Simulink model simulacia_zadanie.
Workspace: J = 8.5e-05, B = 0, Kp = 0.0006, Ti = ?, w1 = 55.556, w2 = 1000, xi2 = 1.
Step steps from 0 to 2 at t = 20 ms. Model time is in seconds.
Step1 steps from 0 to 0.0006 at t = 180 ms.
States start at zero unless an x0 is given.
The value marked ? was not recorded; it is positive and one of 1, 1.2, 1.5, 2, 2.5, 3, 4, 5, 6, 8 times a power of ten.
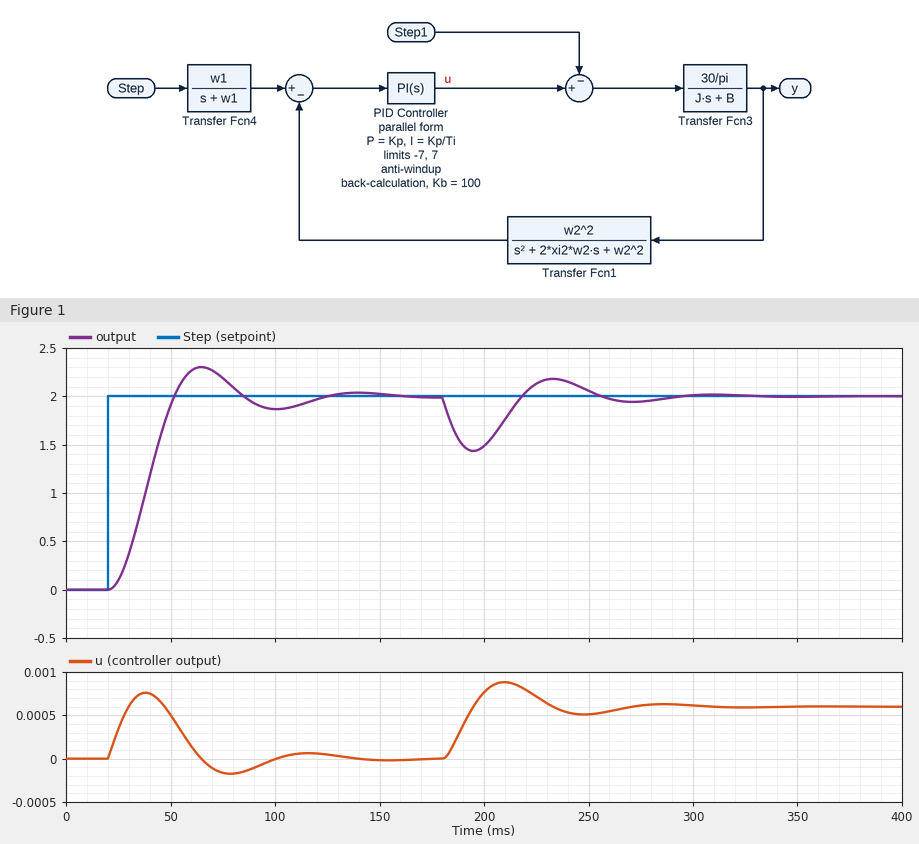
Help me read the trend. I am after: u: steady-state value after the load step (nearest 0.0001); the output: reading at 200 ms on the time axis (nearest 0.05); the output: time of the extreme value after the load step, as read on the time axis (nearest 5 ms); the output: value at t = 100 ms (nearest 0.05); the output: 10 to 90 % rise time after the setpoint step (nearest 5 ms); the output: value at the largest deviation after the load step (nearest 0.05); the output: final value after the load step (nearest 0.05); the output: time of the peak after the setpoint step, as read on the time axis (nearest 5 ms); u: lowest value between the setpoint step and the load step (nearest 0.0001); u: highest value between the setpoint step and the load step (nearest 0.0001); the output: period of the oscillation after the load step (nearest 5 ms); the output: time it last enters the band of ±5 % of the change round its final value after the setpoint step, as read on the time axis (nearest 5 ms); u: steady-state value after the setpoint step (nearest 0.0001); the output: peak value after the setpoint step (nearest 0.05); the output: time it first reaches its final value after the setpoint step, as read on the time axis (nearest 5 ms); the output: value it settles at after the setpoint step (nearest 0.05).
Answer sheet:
0.0006
1.50
195 ms
1.85
20 ms
1.45
2.00
65 ms
-0.0002
0.0008
75 ms
110 ms
0.0000
2.30
50 ms
2.00
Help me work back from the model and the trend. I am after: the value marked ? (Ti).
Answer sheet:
0.01
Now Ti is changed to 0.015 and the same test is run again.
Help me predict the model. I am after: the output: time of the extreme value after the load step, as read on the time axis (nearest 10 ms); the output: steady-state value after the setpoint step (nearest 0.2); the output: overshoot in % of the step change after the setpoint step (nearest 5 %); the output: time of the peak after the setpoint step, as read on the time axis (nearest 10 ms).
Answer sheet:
200 ms
2.0
15 %
70 ms
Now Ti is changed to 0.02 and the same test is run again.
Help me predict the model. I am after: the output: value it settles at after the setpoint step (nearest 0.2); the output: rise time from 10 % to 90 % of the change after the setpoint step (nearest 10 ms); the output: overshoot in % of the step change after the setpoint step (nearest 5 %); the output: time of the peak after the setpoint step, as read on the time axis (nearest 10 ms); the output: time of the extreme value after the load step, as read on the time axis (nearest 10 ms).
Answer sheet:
2.0
30 ms
15 %
80 ms
200 ms
